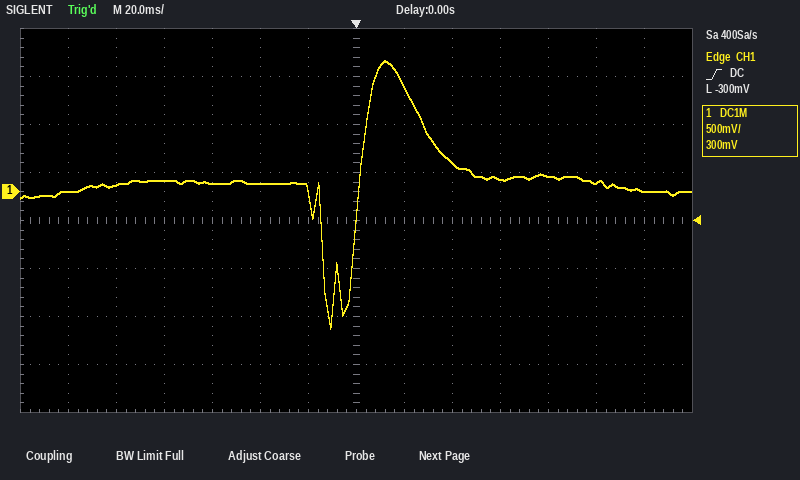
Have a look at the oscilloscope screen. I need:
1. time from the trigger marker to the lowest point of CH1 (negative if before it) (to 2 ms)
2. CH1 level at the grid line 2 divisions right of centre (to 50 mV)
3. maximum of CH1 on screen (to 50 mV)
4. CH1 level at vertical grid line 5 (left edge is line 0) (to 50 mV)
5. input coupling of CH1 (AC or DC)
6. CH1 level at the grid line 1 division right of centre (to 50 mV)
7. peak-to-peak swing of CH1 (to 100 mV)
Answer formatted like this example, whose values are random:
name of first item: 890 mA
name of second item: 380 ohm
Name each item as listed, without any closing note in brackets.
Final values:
time from the trigger marker to the lowest point of CH1 (negative if before it): -10 ms
CH1 level at the grid line 2 divisions right of centre: 300 mV
maximum of CH1 on screen: 1.35 V
CH1 level at vertical grid line 5 (left edge is line 0): 100 mV
input coupling of CH1: DC
CH1 level at the grid line 1 division right of centre: 1.10 V
peak-to-peak swing of CH1: 2.80 V
